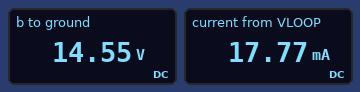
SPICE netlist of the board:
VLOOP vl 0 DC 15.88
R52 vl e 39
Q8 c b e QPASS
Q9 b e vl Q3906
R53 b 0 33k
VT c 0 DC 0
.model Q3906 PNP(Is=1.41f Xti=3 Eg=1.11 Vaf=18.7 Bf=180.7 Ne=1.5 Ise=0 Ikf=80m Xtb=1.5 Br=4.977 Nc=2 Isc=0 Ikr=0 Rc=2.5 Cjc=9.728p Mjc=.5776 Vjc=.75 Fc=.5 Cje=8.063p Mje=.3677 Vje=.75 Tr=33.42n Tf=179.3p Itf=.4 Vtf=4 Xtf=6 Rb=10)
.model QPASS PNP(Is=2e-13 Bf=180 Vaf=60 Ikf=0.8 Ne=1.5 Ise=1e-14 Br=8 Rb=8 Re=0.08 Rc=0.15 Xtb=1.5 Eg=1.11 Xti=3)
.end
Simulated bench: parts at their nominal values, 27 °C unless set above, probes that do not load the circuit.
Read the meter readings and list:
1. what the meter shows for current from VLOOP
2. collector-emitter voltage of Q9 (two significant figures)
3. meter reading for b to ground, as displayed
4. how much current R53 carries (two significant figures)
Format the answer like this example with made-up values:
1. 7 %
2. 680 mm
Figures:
1. 17.77 mA
2. -1.3 V
3. 14.55 V
4. 440 µA
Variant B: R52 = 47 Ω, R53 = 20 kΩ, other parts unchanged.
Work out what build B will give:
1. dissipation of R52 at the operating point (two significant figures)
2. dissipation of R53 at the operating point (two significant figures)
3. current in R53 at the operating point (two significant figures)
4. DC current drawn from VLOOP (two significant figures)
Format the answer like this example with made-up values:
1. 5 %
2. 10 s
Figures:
1. 10 mW
2. 11 mW
3. 730 µA
4. 15 mA
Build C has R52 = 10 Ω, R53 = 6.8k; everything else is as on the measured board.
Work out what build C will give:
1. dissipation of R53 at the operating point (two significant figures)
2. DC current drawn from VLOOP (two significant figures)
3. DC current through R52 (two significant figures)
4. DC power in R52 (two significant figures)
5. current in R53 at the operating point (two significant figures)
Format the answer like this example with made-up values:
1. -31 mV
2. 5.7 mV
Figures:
1. 31 mW
2. 74 mA
3. 72 mA
4. 52 mW
5. 2.1 mA
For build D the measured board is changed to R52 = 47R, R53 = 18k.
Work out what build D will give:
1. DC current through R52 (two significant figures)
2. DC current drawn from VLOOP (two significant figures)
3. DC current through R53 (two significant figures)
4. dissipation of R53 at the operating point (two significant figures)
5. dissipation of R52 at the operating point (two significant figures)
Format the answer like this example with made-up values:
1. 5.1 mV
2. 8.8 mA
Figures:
1. 15 mA
2. 16 mA
3. 810 µA
4. 12 mW
5. 10 mW
